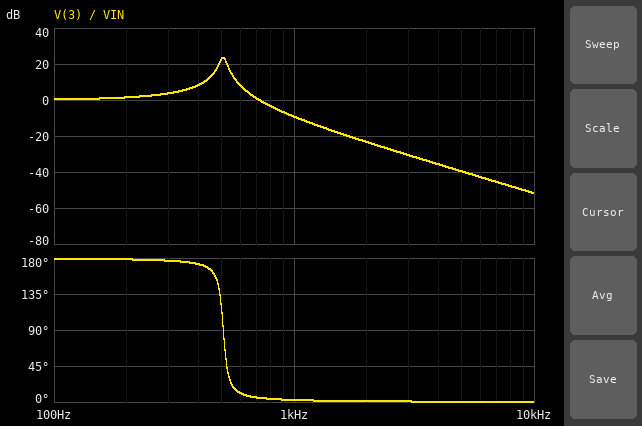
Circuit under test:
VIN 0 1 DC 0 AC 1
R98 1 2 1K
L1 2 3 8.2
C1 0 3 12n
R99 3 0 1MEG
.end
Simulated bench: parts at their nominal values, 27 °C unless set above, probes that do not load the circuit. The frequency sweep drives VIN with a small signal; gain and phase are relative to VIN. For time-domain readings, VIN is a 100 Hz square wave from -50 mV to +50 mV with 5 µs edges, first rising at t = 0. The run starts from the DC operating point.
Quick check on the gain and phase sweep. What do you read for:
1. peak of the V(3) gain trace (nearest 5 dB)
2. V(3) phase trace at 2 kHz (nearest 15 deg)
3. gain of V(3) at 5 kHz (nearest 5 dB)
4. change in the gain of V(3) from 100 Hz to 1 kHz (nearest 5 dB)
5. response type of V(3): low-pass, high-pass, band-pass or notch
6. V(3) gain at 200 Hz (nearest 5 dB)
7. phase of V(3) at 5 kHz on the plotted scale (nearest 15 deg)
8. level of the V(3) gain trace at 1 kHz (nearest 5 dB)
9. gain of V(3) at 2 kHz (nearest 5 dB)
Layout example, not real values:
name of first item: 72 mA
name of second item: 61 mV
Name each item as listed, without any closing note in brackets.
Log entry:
peak of the V(3) gain trace: 25 dB
V(3) phase trace at 2 kHz: 0 deg
gain of V(3) at 5 kHz: -40 dB
change in the gain of V(3) from 100 Hz to 1 kHz: -10 dB
response type of V(3): low-pass, high-pass, band-pass or notch: low-pass
V(3) gain at 200 Hz: 0 dB
phase of V(3) at 5 kHz on the plotted scale: 0 deg
level of the V(3) gain trace at 1 kHz: -10 dB
gain of V(3) at 2 kHz: -25 dB
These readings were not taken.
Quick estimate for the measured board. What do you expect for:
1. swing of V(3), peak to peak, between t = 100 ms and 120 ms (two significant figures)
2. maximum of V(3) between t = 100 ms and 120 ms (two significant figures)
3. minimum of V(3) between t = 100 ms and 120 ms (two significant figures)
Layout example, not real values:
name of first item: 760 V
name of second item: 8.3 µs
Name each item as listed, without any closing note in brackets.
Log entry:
swing of V(3), peak to peak, between t = 100 ms and 120 ms: 520 mV
maximum of V(3) between t = 100 ms and 120 ms: 260 mV
minimum of V(3) between t = 100 ms and 120 ms: -260 mV
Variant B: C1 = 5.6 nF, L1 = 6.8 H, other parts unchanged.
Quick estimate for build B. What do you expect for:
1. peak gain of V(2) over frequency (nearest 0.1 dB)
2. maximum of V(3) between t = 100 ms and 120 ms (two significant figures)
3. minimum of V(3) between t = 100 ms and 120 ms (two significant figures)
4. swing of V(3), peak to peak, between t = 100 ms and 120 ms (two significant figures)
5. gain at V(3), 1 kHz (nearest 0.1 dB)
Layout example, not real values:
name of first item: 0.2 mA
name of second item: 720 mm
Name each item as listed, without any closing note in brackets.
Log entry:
peak gain of V(2) over frequency: 0 dB
maximum of V(3) between t = 100 ms and 120 ms: 110 mV
minimum of V(3) between t = 100 ms and 120 ms: -110 mV
swing of V(3), peak to peak, between t = 100 ms and 120 ms: 230 mV
gain at V(3), 1 kHz: 5.9 dB
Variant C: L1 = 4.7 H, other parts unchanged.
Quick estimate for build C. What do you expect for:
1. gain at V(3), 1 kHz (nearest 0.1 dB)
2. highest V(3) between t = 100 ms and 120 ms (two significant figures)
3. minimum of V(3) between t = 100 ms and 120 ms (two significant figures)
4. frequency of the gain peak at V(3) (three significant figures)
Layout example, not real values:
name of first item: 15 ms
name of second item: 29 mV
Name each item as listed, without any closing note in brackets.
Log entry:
gain at V(3), 1 kHz: -1.8 dB
highest V(3) between t = 100 ms and 120 ms: 160 mV
minimum of V(3) between t = 100 ms and 120 ms: -160 mV
frequency of the gain peak at V(3): 670 Hz
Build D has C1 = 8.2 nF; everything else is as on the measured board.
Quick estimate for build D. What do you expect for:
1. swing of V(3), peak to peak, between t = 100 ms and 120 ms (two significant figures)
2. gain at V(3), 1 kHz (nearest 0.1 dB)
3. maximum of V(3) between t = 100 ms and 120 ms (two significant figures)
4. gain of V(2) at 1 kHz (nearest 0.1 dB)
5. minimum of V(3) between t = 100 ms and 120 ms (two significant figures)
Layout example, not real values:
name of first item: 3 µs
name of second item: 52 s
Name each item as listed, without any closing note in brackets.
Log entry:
swing of V(3), peak to peak, between t = 100 ms and 120 ms: 220 mV
gain at V(3), 1 kHz: -4.4 dB
maximum of V(3) between t = 100 ms and 120 ms: 110 mV
gain of V(2) at 1 kHz: 0 dB
minimum of V(3) between t = 100 ms and 120 ms: -110 mV
